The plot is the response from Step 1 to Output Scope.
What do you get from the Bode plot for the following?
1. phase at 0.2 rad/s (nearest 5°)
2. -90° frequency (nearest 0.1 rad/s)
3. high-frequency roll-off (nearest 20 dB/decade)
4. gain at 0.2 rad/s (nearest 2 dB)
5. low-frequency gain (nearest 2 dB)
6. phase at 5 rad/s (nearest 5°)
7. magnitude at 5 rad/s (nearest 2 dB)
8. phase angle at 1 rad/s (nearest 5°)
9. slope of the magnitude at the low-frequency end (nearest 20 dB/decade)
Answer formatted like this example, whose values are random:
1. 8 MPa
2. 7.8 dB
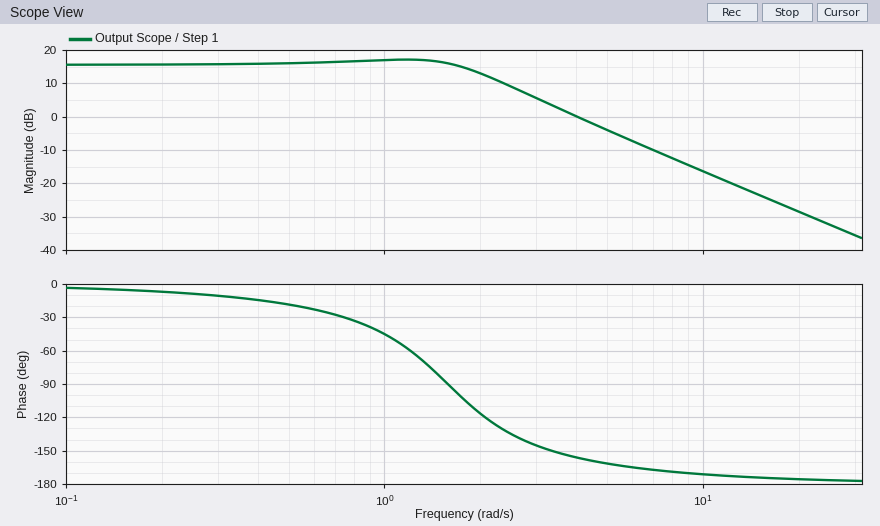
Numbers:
1. -5°
2. 1.6 rad/s
3. -40 dB/decade
4. 16 dB
5. 16 dB
6. -160°
7. -4 dB
8. -45°
9. 0 dB/decade
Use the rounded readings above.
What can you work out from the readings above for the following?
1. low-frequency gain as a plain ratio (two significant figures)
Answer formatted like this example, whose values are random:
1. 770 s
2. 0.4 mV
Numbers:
1. 6.3
